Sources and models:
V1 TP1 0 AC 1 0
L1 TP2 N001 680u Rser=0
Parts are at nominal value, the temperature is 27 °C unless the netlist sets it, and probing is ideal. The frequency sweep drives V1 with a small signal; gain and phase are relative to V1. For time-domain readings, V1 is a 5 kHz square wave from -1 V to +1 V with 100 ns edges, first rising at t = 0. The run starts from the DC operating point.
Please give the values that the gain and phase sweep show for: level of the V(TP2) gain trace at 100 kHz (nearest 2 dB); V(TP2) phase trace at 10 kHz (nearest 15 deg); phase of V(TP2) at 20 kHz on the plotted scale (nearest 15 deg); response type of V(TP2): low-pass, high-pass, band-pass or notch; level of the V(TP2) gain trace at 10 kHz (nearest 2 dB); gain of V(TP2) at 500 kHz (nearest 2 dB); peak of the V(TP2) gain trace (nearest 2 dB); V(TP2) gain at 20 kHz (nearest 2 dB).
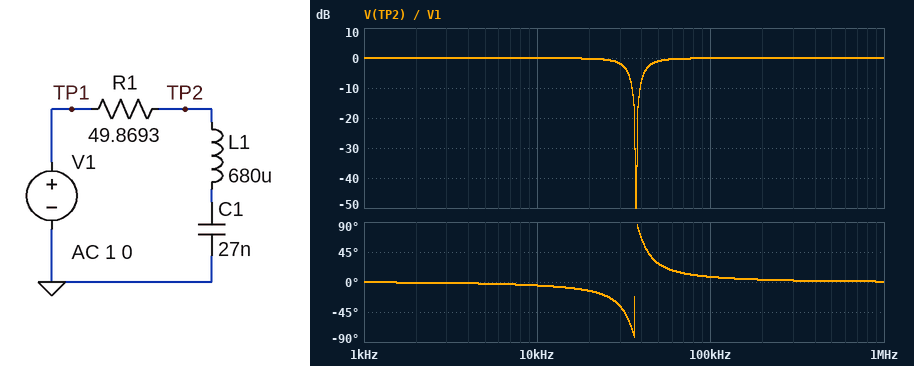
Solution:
0 dB
0 deg
-15 deg
notch
0 dB
0 dB
0 dB
0 dB
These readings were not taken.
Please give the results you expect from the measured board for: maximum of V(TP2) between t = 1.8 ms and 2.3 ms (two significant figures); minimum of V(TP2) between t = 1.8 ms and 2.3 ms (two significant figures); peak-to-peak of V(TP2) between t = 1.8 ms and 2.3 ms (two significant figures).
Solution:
1.3 V
-1.3 V
2.6 V
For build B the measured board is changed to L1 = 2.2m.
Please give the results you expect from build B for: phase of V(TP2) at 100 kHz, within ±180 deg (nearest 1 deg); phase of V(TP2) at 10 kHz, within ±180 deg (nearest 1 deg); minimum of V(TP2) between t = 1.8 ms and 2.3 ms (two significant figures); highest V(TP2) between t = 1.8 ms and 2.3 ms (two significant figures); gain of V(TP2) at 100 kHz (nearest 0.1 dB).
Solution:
2 deg
-6 deg
-1.2 V
1.2 V
0 dB
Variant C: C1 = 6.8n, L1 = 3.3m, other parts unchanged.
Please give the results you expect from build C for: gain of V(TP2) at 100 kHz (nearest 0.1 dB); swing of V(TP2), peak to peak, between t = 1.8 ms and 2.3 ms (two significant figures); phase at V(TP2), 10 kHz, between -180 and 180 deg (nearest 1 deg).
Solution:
0 dB
2.3 V
-1 deg
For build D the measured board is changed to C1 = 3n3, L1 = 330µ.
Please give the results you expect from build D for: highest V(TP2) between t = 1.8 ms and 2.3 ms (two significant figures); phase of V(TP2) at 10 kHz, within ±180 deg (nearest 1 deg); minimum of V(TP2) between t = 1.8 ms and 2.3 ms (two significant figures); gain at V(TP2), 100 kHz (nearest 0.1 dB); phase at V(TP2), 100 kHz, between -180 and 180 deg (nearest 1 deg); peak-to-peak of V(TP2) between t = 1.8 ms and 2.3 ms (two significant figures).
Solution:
1.2 V
-1 deg
-1.2 V
-0.1 dB
-10 deg
2.4 V
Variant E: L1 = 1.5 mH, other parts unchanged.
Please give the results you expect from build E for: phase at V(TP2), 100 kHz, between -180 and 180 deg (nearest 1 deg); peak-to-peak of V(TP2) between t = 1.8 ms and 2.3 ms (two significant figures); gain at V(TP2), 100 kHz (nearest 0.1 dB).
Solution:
3 deg
2.6 V
0 dB
